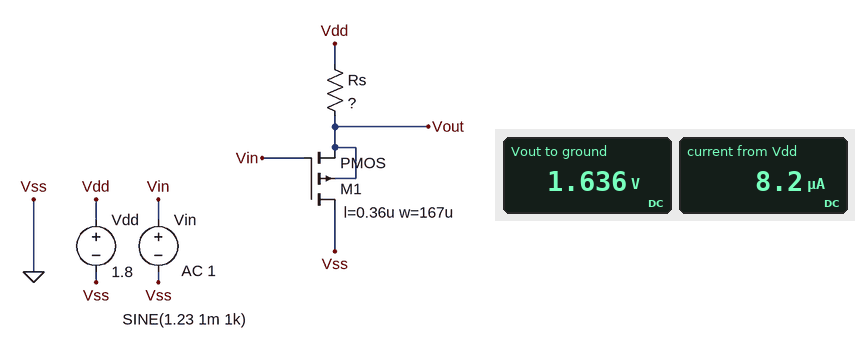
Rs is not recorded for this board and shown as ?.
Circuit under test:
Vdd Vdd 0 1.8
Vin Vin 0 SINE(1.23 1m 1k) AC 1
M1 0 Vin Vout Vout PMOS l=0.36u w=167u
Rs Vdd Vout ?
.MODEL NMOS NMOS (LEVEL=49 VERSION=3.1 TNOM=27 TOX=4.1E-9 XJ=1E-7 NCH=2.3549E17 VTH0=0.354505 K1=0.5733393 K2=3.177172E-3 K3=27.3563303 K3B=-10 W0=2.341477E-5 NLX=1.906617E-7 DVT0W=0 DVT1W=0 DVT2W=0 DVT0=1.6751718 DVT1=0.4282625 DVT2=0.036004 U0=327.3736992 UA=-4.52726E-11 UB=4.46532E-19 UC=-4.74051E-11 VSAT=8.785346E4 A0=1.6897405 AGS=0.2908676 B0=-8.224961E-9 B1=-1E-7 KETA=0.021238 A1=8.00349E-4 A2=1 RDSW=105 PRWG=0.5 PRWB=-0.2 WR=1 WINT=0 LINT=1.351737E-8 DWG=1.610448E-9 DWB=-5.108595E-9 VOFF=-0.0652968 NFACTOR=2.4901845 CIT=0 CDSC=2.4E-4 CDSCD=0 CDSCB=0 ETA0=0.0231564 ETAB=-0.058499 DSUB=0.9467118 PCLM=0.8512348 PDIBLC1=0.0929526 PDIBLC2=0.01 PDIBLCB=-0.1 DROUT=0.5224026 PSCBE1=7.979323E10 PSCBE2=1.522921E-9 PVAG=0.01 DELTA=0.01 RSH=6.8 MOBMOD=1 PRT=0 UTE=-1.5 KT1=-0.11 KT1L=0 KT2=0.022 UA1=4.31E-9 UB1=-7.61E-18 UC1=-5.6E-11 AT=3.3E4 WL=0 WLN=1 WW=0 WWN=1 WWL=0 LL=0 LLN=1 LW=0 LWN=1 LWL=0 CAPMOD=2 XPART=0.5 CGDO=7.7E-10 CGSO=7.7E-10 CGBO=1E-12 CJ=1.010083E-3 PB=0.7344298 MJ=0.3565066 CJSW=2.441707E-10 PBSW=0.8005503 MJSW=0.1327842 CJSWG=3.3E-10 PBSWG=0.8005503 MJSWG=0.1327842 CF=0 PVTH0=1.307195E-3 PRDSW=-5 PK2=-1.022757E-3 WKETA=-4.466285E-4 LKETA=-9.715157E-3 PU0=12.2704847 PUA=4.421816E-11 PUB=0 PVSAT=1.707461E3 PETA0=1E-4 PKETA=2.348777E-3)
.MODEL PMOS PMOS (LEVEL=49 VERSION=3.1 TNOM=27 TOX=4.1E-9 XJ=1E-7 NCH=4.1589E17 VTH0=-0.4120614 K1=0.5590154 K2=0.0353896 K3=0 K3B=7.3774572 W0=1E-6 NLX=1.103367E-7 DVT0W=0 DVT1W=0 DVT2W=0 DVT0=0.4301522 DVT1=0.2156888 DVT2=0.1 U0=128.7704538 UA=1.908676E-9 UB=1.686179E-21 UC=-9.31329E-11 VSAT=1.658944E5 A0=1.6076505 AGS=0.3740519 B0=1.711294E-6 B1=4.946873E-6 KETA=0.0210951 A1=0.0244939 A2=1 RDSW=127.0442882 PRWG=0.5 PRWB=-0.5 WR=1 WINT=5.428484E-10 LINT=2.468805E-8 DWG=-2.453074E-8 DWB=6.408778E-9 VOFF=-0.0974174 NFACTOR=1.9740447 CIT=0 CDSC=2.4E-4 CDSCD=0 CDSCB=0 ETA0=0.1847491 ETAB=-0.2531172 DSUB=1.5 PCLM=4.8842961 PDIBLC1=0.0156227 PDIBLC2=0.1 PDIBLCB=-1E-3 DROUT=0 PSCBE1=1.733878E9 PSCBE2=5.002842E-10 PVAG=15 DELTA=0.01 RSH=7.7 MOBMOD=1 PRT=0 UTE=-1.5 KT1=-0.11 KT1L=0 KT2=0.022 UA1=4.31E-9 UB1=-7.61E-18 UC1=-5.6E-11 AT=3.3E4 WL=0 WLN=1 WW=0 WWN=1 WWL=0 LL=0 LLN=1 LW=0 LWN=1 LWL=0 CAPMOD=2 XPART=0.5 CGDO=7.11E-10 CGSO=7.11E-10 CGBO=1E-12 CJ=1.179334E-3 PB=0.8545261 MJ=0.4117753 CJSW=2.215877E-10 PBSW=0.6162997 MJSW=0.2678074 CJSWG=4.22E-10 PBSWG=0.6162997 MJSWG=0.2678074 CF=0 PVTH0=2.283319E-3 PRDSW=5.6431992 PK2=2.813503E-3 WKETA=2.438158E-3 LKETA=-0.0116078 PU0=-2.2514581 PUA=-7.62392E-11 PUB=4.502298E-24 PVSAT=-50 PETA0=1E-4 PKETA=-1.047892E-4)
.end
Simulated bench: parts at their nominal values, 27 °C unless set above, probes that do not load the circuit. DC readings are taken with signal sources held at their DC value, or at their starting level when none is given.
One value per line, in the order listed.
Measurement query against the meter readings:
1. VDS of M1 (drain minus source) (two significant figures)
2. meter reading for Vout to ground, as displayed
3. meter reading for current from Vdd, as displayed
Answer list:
-1.6 V
1.636 V
8.2 µA
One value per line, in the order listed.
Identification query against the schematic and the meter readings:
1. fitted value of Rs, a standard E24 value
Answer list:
20 kΩ
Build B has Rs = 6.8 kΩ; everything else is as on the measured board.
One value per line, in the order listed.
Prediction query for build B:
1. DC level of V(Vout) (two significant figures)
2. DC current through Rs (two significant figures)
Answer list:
1.7 V
19 µA
